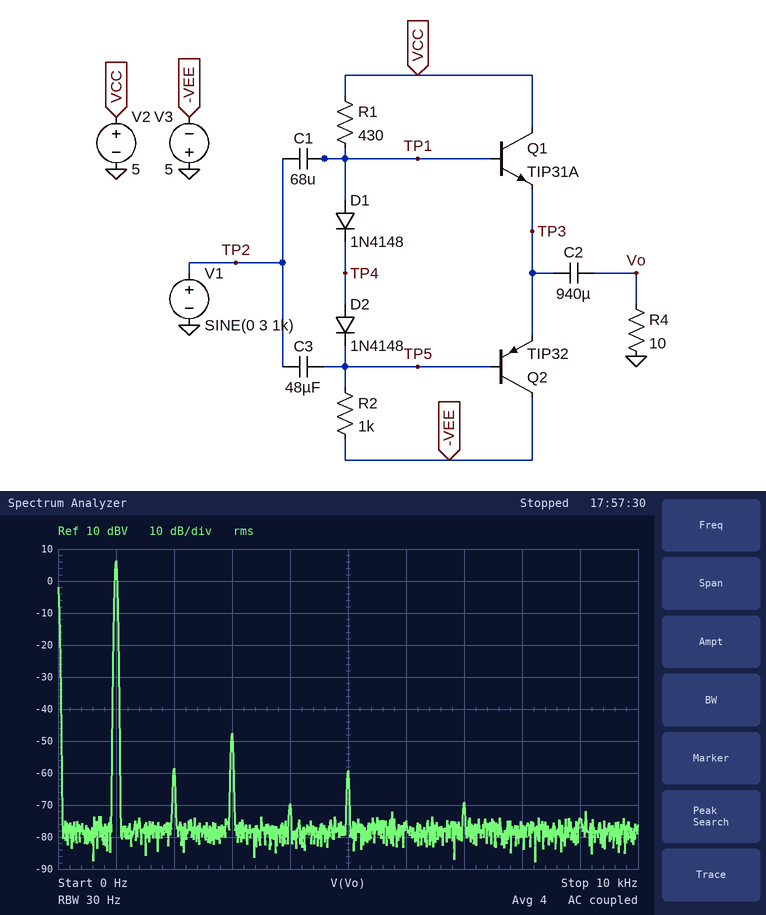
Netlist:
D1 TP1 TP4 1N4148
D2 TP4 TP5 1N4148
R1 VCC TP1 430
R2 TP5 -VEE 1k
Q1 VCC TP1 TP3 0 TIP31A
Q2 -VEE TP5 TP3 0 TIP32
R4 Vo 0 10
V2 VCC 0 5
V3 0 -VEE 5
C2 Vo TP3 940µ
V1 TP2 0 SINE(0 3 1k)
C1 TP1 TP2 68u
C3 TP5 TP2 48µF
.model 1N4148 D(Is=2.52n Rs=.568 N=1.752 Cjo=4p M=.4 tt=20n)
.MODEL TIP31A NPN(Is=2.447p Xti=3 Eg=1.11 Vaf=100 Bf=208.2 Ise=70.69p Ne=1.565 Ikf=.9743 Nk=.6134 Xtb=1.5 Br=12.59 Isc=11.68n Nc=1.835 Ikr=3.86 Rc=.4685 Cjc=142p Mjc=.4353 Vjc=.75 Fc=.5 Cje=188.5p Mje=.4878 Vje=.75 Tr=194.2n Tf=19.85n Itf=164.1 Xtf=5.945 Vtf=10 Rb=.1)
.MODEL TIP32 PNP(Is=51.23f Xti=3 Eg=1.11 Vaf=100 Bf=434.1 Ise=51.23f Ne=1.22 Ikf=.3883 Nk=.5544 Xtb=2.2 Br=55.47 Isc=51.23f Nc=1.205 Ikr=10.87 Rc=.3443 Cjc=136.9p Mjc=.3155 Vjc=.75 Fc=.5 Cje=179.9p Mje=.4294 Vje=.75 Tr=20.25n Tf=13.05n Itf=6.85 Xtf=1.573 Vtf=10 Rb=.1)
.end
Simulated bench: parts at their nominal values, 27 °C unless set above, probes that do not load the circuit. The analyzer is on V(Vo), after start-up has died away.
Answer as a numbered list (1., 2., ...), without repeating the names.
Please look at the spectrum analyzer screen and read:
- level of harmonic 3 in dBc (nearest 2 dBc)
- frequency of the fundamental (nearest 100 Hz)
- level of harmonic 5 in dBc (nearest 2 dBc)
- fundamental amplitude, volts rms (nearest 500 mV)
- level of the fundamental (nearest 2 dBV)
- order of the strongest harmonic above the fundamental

1. -54 dBc
2. 1.0 kHz
3. -66 dBc
4. 2.0 V
5. 6 dBV
6. 3
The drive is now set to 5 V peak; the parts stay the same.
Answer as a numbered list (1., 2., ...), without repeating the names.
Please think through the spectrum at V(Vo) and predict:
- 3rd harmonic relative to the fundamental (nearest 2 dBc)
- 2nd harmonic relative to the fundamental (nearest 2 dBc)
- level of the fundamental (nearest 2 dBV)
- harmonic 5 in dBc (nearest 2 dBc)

1. -44 dBc
2. -46 dBc
3. 10 dBV
4. -46 dBc
